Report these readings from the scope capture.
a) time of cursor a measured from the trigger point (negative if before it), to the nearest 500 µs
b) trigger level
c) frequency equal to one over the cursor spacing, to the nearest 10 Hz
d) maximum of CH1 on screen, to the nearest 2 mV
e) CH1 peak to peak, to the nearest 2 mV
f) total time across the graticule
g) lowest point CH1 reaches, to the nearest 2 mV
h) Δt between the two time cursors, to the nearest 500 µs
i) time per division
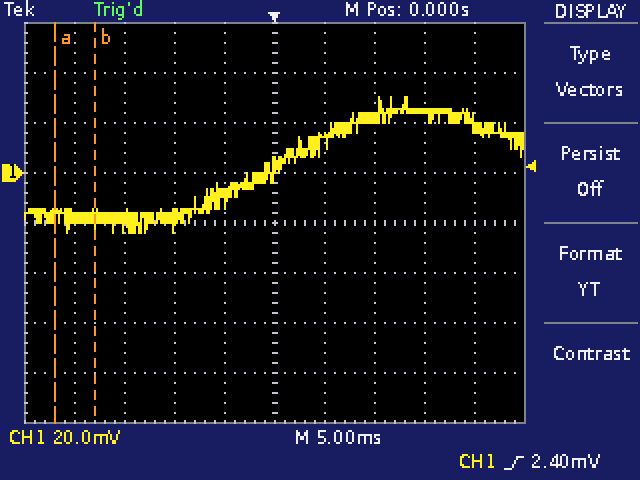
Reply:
-22.0 ms
2.40 mV
250 Hz
30 mV
54 mV
50 ms
-24 mV
4.0 ms
5 ms
